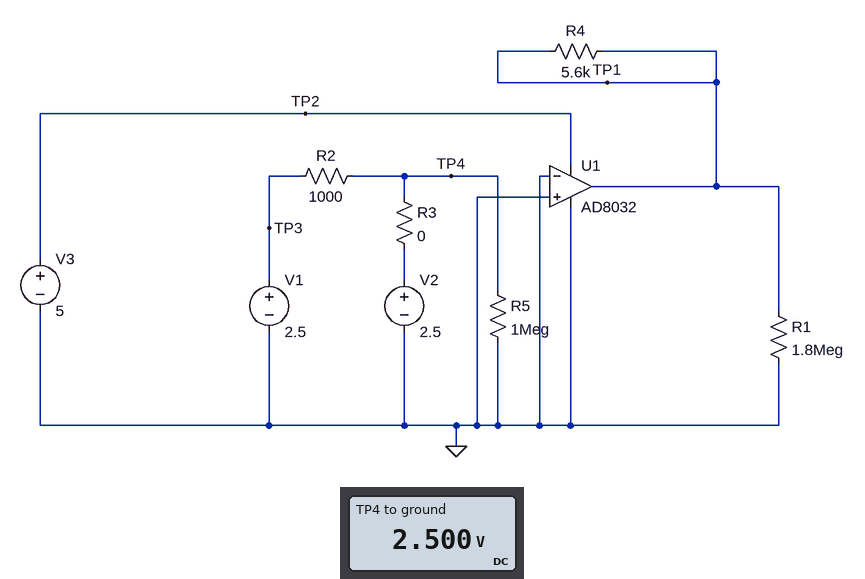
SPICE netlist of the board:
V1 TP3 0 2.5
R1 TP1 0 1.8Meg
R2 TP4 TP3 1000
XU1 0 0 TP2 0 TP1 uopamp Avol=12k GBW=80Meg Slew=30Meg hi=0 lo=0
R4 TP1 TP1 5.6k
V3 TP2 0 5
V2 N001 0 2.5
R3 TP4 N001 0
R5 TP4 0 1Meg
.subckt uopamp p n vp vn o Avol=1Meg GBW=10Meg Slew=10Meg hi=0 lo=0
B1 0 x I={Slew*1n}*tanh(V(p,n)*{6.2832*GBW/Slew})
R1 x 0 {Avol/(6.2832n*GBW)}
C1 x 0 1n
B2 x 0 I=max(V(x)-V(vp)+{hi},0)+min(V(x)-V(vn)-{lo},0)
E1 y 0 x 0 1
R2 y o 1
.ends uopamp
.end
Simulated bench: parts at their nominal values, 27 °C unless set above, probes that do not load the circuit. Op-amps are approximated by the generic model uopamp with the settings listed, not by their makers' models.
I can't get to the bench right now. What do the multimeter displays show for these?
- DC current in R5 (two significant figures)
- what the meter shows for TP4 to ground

2.5 µA
2.500 V
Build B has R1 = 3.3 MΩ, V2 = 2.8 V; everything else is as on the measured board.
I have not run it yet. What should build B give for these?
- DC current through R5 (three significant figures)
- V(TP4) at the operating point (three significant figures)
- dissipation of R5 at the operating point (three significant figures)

2.80 µA
2.80 V
7.84 µW
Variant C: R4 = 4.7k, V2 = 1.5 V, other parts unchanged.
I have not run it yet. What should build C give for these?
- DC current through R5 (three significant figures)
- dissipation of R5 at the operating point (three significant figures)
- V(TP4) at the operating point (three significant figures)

1.50 µA
2.25 µW
1.50 V
